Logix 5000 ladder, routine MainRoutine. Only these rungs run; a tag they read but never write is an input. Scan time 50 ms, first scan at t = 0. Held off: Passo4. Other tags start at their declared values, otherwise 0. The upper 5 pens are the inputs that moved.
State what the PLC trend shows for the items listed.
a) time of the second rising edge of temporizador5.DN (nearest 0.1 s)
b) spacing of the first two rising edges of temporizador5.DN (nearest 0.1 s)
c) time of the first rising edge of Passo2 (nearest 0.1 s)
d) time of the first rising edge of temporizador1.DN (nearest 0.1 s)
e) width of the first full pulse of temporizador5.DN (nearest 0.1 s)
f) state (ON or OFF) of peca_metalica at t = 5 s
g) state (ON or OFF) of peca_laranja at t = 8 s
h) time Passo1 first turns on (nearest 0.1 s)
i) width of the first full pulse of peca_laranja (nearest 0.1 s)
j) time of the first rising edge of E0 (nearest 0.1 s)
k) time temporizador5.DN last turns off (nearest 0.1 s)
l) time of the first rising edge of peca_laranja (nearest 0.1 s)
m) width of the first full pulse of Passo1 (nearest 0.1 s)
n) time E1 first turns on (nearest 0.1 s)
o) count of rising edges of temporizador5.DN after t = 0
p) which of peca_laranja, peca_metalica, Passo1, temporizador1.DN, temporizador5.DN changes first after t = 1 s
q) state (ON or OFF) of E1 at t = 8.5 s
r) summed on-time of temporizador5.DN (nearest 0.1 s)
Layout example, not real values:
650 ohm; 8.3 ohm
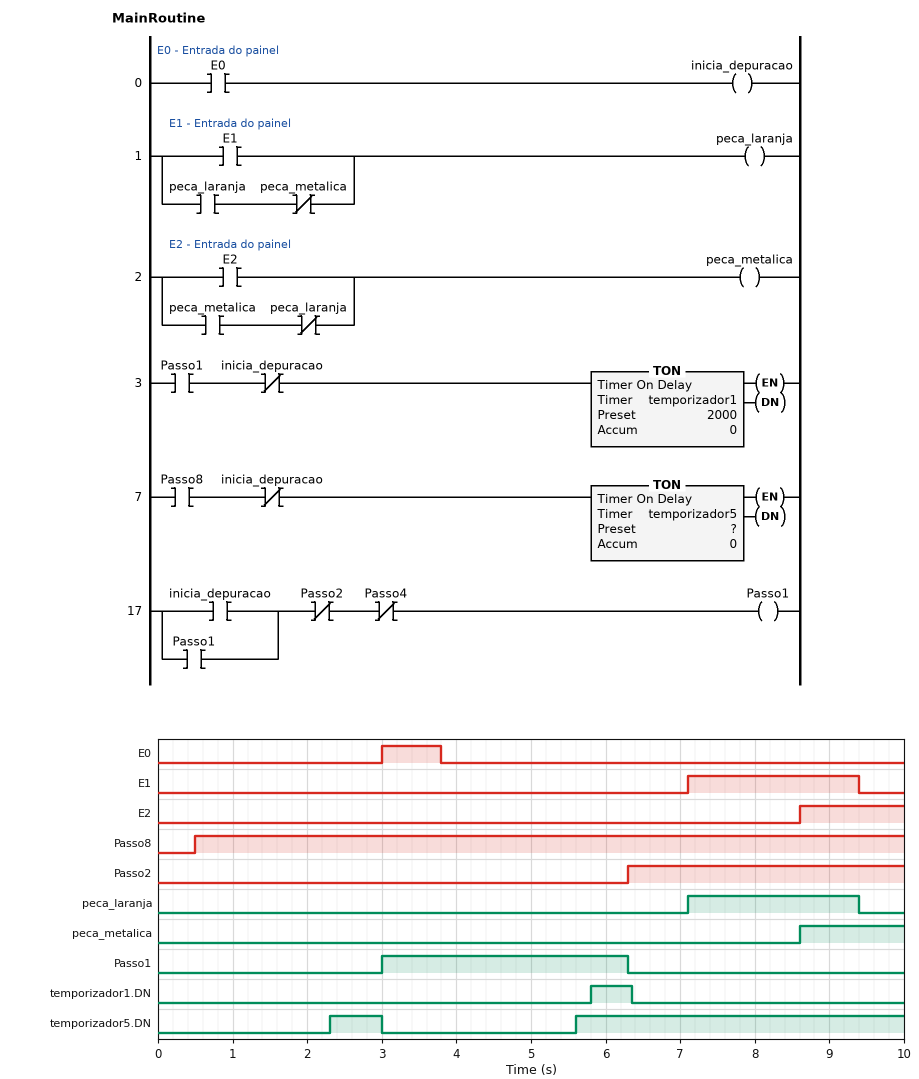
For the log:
5.6 s; 3.3 s; 6.3 s; 5.8 s; 0.7 s; OFF; ON; 3.0 s; 2.3 s; 3.0 s; 3.0 s; 7.1 s; 3.3 s; 7.1 s; 2; temporizador5.DN; ON; 5.1 s
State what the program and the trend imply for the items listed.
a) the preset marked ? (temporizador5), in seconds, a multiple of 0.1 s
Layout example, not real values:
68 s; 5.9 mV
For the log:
1.8 s
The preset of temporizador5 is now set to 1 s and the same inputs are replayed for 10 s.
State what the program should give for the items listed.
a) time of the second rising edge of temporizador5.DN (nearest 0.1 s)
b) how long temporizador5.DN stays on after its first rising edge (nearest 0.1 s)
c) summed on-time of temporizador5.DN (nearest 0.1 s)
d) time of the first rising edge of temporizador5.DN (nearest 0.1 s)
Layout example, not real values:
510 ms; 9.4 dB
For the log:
4.8 s; 1.5 s; 6.7 s; 1.5 s
